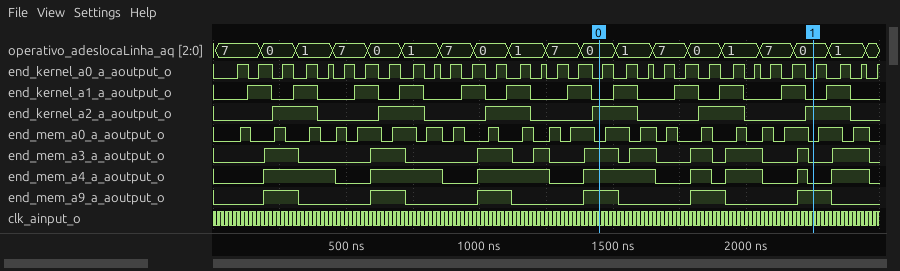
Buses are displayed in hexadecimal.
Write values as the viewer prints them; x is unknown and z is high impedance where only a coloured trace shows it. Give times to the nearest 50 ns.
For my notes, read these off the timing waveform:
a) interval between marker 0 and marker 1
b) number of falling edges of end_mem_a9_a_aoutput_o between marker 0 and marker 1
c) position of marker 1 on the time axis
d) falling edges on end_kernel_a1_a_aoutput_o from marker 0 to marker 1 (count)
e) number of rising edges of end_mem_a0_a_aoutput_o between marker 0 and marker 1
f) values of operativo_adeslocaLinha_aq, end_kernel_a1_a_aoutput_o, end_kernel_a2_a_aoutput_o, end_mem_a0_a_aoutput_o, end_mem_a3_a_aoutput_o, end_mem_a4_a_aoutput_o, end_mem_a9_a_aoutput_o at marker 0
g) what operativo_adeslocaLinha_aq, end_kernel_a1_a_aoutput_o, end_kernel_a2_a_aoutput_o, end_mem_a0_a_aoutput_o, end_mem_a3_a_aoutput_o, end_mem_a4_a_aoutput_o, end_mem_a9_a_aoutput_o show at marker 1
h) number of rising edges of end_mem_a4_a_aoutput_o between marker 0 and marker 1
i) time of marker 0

800 ns
2
2250 ns
4
7
operativo_adeslocaLinha_aq=0, end_kernel_a1_a_aoutput_o=0, end_kernel_a2_a_aoutput_o=1, end_mem_a0_a_aoutput_o=0, end_mem_a3_a_aoutput_o=1, end_mem_a4_a_aoutput_o=1, end_mem_a9_a_aoutput_o=1
operativo_adeslocaLinha_aq=0, end_kernel_a1_a_aoutput_o=0, end_kernel_a2_a_aoutput_o=1, end_mem_a0_a_aoutput_o=0, end_mem_a3_a_aoutput_o=0, end_mem_a4_a_aoutput_o=0, end_mem_a9_a_aoutput_o=1
3
1450 ns
